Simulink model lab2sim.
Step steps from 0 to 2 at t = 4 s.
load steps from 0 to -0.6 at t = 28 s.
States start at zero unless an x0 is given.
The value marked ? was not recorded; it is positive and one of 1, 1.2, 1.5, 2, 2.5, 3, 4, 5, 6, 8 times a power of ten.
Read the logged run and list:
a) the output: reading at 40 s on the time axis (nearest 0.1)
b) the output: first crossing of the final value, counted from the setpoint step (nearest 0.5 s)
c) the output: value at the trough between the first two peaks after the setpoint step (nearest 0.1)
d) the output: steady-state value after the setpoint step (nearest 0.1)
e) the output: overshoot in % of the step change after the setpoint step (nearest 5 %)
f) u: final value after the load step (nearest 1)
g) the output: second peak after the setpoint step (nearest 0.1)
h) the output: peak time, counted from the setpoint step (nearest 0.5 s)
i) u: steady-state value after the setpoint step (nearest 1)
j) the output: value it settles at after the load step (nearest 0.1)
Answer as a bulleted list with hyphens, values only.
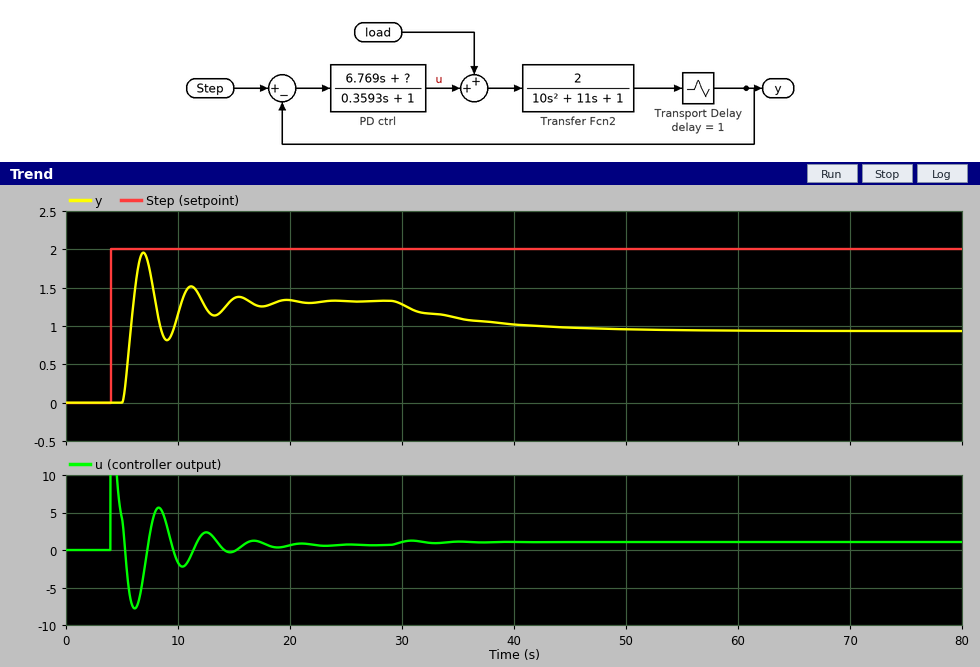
- 1.0
- 2.0 s
- 0.8
- 1.3
- 45 %
- 1
- 1.5
- 3.0 s
- 1
- 0.9
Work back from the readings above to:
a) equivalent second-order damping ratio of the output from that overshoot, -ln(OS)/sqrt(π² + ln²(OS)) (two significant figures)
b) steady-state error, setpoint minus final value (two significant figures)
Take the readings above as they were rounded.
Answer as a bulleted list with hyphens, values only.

- 0.25
- 0.70
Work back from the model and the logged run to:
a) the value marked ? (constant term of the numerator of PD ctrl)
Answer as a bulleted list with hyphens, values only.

- 1
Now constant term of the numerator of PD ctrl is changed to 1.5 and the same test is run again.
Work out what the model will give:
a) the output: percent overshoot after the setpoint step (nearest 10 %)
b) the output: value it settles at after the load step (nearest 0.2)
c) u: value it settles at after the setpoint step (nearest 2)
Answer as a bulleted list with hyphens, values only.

- 40 %
- 1.2
- 0
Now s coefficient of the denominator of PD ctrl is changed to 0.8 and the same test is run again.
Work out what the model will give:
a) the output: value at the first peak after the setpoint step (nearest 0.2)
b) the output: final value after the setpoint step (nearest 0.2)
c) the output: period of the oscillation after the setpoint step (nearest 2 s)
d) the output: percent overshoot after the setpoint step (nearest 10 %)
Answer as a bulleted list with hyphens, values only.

- 1.8
- 1.4
- 6 s
- 40 %
